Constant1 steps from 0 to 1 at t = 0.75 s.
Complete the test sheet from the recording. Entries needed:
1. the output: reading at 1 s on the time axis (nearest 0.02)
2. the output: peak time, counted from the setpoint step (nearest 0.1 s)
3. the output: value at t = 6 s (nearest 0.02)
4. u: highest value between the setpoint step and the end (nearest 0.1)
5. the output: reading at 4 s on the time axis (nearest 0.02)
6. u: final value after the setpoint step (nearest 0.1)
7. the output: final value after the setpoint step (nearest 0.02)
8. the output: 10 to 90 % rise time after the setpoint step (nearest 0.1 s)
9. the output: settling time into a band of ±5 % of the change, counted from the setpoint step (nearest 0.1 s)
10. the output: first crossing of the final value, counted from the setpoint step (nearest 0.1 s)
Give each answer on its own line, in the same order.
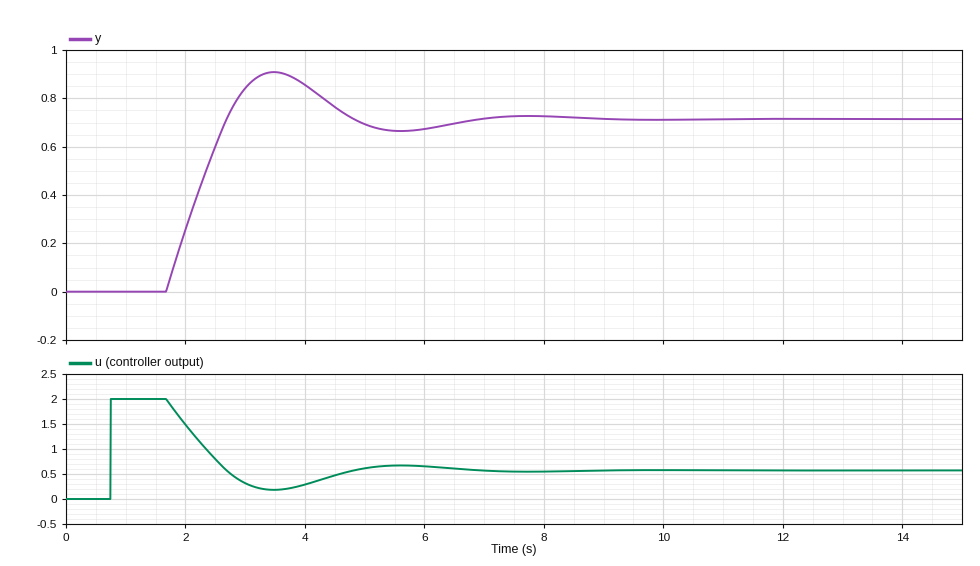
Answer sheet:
0.00
2.7 s
0.68
2.0
0.86
0.6
0.72
0.8 s
5.4 s
1.9 s
